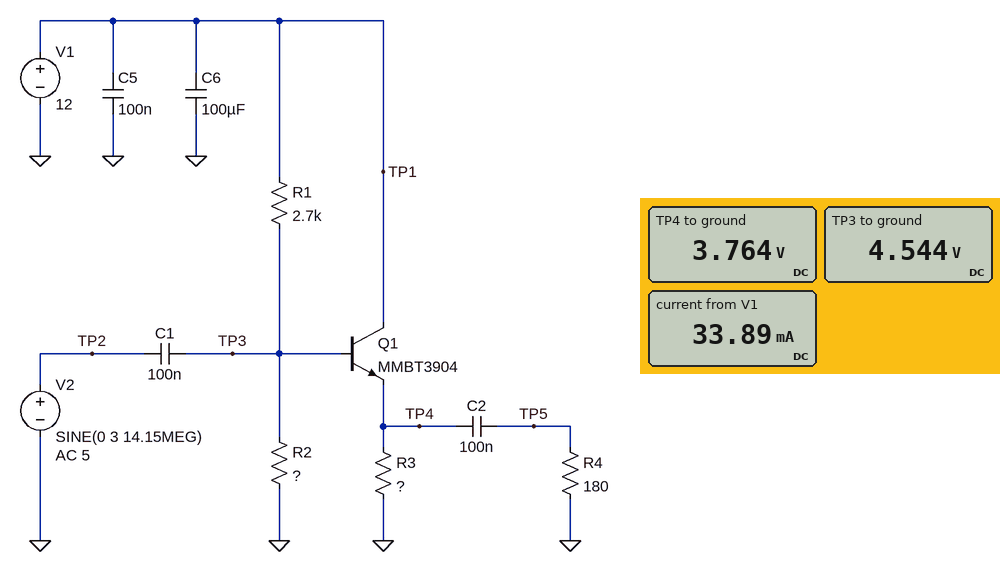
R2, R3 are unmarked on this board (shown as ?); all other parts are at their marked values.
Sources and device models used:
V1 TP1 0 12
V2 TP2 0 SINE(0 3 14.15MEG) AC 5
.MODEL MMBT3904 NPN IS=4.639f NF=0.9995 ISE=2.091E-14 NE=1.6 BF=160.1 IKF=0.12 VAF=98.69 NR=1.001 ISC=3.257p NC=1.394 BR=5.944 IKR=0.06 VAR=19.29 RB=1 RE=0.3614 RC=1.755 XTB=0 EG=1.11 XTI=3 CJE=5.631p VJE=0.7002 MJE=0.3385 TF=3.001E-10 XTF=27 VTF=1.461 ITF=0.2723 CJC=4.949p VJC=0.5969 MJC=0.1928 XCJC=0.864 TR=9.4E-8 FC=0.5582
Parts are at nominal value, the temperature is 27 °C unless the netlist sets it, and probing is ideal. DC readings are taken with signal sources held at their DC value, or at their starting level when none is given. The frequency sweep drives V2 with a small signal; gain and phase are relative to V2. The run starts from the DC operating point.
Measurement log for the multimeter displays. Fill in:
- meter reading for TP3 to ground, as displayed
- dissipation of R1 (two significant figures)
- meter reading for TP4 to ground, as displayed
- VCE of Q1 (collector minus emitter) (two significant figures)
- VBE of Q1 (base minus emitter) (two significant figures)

4.544 V
21 mW
3.764 V
8.2 V
780 mV
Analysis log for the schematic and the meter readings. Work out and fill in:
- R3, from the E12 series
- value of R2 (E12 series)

120 Ω
1.8 kΩ
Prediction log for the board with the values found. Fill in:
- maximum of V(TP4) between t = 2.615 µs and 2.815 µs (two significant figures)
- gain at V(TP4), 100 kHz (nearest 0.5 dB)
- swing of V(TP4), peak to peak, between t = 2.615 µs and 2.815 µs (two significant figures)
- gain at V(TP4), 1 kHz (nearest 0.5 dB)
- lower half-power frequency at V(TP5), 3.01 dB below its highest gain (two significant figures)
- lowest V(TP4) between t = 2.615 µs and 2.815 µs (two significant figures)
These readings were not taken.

6.7 V
0 dB
5.3 V
-5.5 dB
9.1 kHz
1.4 V
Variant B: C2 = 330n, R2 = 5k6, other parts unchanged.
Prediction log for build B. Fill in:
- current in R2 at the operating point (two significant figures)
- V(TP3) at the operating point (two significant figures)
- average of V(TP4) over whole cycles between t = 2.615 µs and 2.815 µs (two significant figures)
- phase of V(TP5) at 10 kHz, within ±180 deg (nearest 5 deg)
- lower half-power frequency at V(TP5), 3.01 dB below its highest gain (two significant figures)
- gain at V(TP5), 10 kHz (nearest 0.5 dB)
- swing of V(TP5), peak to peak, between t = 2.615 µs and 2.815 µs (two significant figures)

1.3 mA
7.2 V
6.4 V
20 deg
3.1 kHz
-0.5 dB
5.9 V
